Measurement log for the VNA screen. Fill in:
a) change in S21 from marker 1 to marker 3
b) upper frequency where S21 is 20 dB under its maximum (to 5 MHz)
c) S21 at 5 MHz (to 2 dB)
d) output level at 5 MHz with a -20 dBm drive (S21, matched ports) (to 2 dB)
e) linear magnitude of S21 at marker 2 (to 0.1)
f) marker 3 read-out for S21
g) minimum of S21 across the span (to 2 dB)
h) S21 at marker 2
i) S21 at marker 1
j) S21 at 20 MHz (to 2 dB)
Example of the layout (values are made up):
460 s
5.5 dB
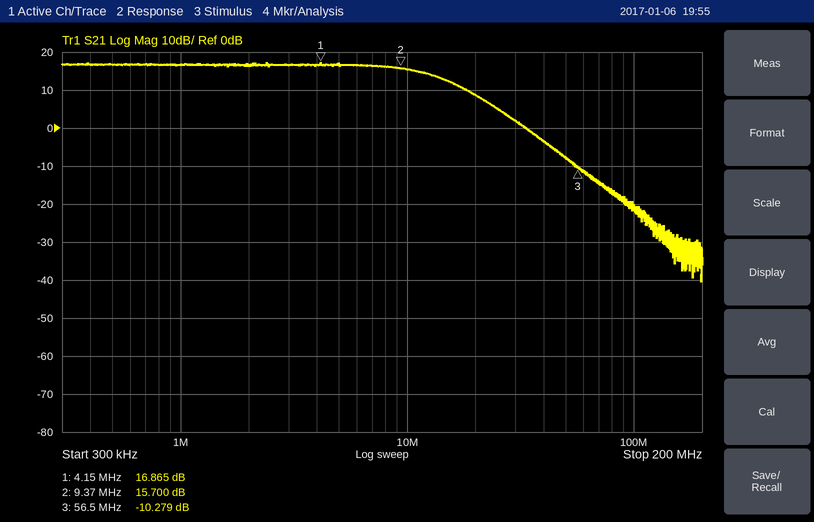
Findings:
-27.144 dB
40 MHz
16 dB
-4 dBm
6.1
-10.279 dB
-40 dB
15.700 dB
16.865 dB
8 dB
